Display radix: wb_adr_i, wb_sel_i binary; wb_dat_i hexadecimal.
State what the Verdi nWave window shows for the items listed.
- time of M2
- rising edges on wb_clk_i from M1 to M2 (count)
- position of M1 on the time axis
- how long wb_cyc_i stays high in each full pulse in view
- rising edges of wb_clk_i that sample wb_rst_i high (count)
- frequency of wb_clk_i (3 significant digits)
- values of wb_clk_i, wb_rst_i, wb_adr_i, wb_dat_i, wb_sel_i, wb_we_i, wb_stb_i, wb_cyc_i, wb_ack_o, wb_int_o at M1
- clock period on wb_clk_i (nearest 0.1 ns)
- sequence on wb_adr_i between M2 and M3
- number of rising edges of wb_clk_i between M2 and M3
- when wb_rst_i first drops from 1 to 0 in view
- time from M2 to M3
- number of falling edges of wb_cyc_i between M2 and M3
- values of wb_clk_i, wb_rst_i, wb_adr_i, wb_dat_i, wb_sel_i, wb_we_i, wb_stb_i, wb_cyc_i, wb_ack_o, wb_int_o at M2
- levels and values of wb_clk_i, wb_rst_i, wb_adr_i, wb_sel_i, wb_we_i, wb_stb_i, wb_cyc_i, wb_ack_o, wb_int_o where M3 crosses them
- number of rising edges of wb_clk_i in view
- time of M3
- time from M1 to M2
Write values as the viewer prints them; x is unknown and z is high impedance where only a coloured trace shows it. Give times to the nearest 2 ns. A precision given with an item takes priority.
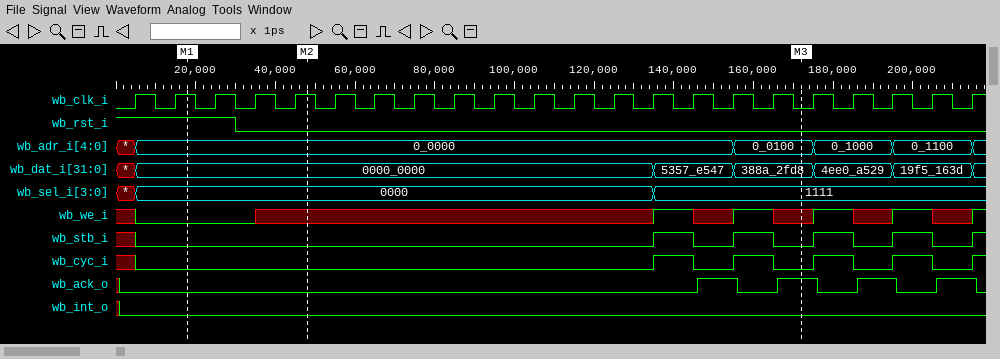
48 ns
3
18 ns
10 ns, 10 ns, 10 ns, 10 ns
3
100 MHz
wb_clk_i=1, wb_rst_i=1, wb_adr_i=0_0000, wb_dat_i=0000_0000, wb_sel_i=0000, wb_we_i=0, wb_stb_i=0, wb_cyc_i=0, wb_ack_o=0, wb_int_o=0
10 ns
0_0000, 0_0100
12
30 ns
124 ns
2
wb_clk_i=1, wb_rst_i=0, wb_adr_i=0_0000, wb_dat_i=0000_0000, wb_sel_i=0000, wb_we_i=x, wb_stb_i=0, wb_cyc_i=0, wb_ack_o=0, wb_int_o=0
wb_clk_i=0, wb_rst_i=0, wb_adr_i=0_0100, wb_sel_i=1111, wb_we_i=x, wb_stb_i=0, wb_cyc_i=0, wb_ack_o=1, wb_int_o=0
22
172 ns
30 ns
